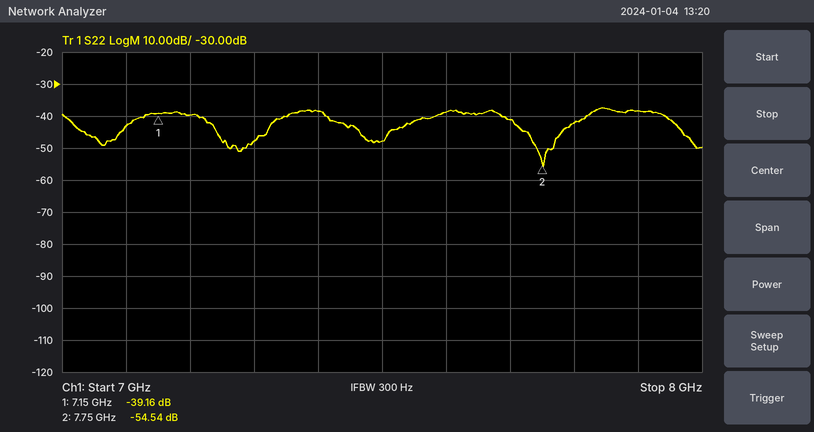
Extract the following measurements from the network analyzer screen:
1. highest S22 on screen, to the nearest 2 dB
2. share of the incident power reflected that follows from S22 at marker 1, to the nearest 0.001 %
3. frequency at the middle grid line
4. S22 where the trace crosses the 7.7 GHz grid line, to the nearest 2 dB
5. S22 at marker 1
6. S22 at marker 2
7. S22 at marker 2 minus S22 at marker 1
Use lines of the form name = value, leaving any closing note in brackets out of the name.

highest S22 on screen, to the nearest 2 dB = -38 dB
share of the incident power reflected that follows from S22 at marker 1, to the nearest 0.001 % = 0.012 %
frequency at the middle grid line = 7.5 GHz
S22 where the trace crosses the 7.7 GHz grid line, to the nearest 2 dB = -42 dB
S22 at marker 1 = -39.16 dB
S22 at marker 2 = -54.54 dB
S22 at marker 2 minus S22 at marker 1 = -15.38 dB
